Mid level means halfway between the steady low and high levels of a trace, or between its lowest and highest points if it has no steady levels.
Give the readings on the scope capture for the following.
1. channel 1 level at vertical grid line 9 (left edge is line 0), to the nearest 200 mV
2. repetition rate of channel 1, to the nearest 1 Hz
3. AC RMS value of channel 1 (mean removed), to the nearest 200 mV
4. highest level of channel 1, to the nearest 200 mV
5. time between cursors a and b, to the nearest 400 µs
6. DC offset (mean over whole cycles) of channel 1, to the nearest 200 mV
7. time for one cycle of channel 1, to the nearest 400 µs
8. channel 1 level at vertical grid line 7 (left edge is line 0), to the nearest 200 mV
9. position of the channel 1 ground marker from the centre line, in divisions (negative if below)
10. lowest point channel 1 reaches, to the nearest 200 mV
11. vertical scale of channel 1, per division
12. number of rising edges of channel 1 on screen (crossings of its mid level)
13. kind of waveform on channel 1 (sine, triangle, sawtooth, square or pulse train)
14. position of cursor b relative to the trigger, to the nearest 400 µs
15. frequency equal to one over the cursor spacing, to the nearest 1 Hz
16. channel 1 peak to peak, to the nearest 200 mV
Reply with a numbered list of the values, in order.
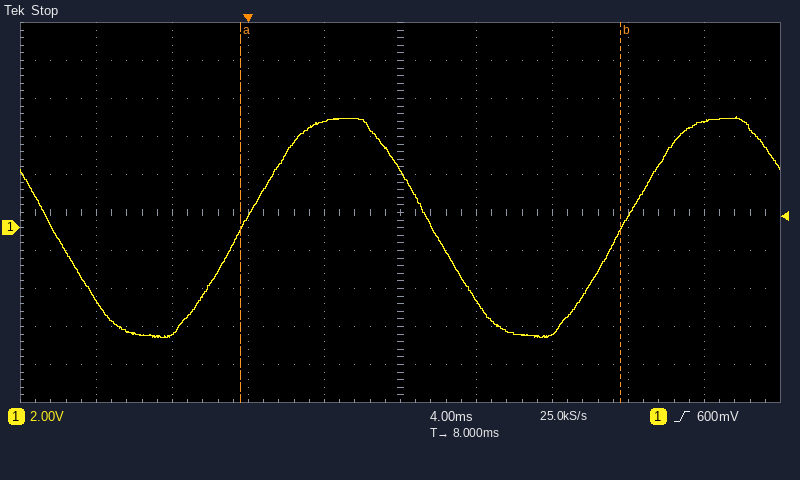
1. 5.6 V
2. 50 Hz
3. 4.2 V
4. 5.8 V
5. 20.0 ms
6. 0.0 V
7. 20.0 ms
8. -5.6 V
9. -0.4 div
10. -5.8 V
11. 2 V
12. 2
13. sine
14. +19.6 ms
15. 50 Hz
16. 11.6 V
